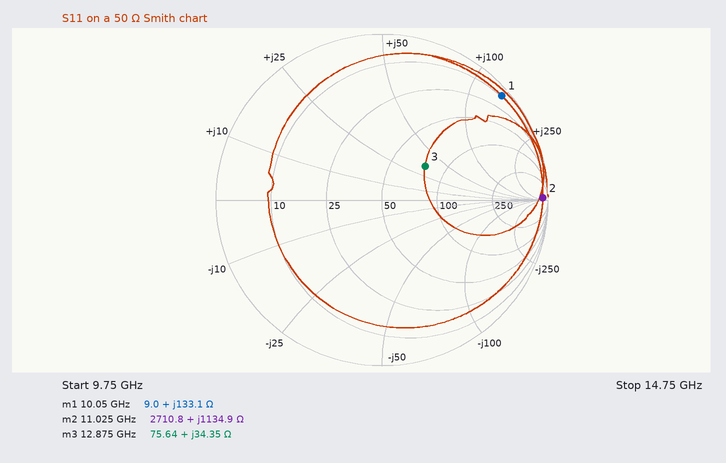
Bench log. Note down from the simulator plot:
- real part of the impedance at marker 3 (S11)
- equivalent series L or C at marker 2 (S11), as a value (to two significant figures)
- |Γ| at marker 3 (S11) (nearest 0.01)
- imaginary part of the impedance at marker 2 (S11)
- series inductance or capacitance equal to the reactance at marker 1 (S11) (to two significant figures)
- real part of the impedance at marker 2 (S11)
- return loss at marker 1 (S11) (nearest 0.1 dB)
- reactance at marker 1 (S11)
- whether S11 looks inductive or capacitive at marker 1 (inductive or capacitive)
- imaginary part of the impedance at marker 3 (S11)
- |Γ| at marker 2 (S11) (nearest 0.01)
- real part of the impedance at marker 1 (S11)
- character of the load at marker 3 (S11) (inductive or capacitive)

75.64 Ω
16 nH
0.33
+1134.9 Ω
2.1 nH
2710.8 Ω
0.4 dB
+133.1 Ω
inductive
+34.35 Ω
0.97
9.0 Ω
inductive
